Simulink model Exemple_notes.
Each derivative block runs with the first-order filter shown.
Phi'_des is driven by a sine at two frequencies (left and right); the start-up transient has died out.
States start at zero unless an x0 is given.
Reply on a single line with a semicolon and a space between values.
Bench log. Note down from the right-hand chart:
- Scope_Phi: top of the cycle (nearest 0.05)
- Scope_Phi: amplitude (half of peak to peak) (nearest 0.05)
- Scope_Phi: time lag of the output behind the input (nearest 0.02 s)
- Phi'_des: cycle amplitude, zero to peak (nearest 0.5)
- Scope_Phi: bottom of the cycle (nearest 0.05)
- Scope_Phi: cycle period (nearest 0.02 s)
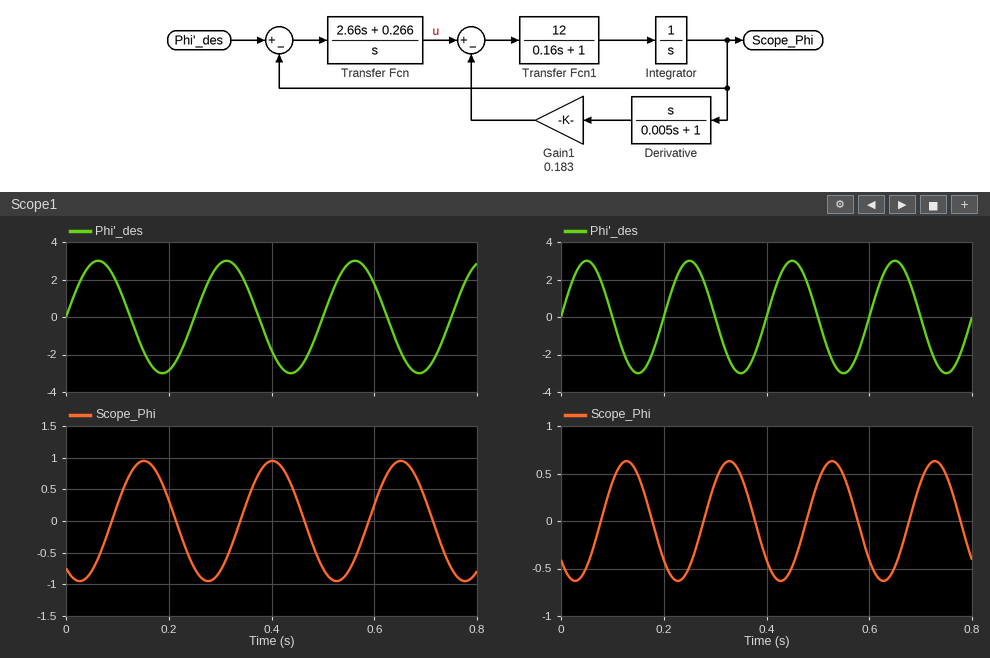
0.65; 0.65; 0.08 s; 3.0; -0.65; 0.20 s
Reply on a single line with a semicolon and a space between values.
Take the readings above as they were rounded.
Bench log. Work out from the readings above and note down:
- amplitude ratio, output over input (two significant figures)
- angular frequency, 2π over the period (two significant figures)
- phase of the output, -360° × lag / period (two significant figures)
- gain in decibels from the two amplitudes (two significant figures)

0.22; 31 rad/s; -140°; -13 dB
